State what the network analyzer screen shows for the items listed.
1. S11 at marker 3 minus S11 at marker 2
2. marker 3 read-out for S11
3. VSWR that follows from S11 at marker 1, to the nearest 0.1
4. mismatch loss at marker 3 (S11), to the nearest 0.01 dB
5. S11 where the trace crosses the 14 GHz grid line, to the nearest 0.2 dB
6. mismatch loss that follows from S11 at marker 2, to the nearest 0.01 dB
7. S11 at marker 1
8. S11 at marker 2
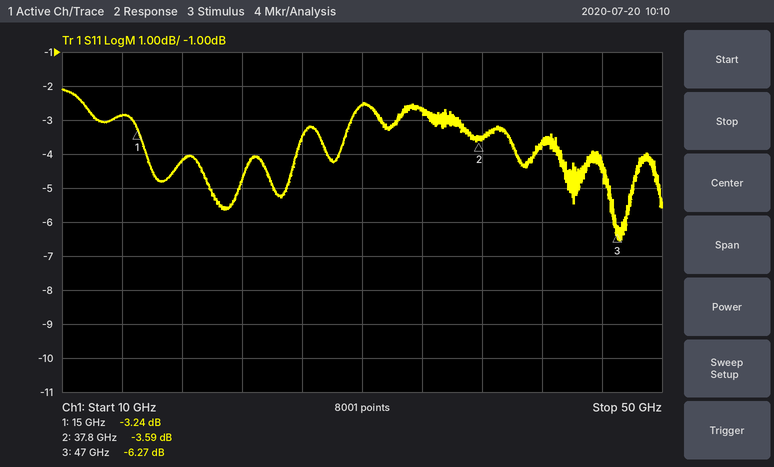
-2.68 dB
-6.27 dB
5.4
1.17 dB
-2.8 dB
2.50 dB
-3.24 dB
-3.59 dB
